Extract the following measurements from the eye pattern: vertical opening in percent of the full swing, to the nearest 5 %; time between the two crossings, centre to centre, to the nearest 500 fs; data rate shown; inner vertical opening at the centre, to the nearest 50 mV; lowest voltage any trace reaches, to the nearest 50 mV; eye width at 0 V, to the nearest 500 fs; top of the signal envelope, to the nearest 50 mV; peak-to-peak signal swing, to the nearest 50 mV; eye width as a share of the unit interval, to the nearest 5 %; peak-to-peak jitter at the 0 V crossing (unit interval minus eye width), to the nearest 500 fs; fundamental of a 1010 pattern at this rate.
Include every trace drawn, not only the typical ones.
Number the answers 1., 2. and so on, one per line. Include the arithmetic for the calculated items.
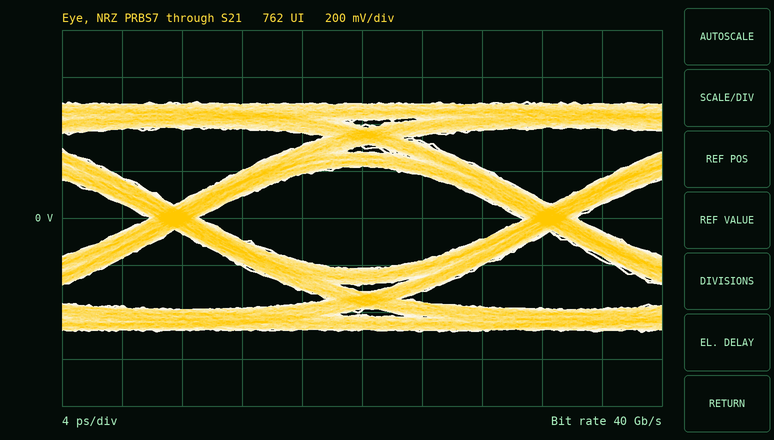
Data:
1. 450 mV / 1.00 V ≈ 45 %
2. 25.0 ps
3. 40 Gb/s
4. 450 mV
5. -500 mV
6. 21.5 ps
7. 500 mV
8. 1.00 V
9. 21.5 ps / 25.0 ps ≈ 86.0 %, so 85 % to the nearest 5 %
10. 3.5 ps
11. 20 GHz
